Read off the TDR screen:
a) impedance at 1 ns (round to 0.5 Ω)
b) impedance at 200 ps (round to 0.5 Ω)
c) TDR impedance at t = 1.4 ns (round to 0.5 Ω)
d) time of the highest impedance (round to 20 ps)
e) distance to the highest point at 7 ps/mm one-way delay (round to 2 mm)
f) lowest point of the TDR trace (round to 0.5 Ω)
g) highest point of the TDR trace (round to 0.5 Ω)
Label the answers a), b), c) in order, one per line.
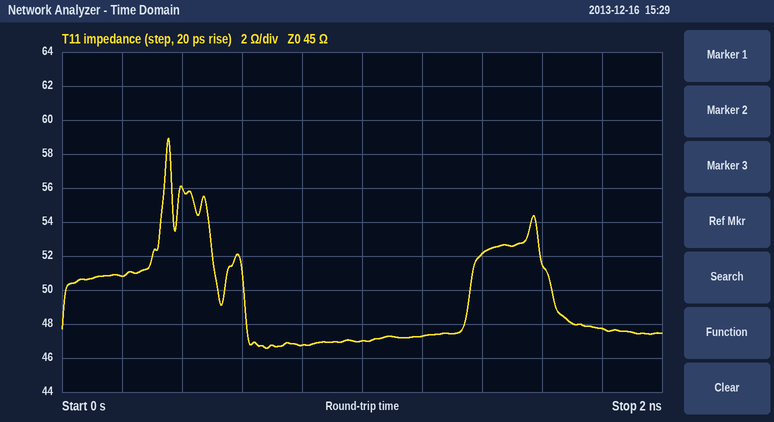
a) 47.0 Ω
b) 51.0 Ω
c) 52.0 Ω
d) 360 ps
e) 26 mm
f) 46.5 Ω
g) 59.0 Ω
